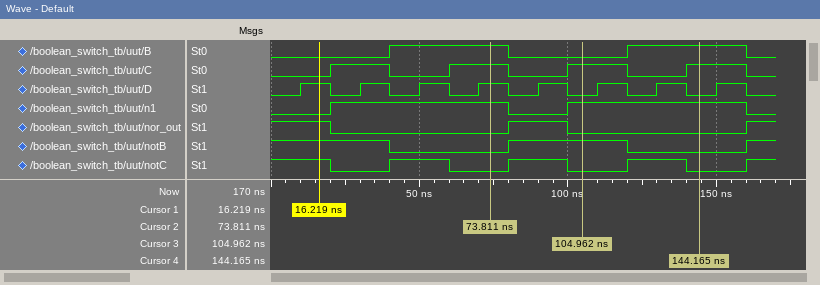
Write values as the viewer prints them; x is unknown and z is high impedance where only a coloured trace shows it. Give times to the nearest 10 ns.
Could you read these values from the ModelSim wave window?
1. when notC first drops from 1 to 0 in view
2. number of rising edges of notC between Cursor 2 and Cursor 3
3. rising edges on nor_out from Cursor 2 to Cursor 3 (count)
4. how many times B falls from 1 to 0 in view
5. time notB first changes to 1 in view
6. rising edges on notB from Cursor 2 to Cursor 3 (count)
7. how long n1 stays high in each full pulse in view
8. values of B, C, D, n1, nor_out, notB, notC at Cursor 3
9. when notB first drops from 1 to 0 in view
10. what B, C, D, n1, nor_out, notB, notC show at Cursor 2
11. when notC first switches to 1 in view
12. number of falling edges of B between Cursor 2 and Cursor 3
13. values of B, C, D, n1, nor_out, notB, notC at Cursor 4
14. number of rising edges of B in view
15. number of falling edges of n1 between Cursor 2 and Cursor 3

20 ns
1
1
2
80 ns
1
60 ns, 60 ns
B=0, C=1, D=0, n1=1, nor_out=0, notB=1, notC=0
40 ns
B=1, C=1, D=1, n1=1, nor_out=0, notB=0, notC=0
40 ns
1
B=1, C=1, D=0, n1=1, nor_out=0, notB=0, notC=0
2
1
